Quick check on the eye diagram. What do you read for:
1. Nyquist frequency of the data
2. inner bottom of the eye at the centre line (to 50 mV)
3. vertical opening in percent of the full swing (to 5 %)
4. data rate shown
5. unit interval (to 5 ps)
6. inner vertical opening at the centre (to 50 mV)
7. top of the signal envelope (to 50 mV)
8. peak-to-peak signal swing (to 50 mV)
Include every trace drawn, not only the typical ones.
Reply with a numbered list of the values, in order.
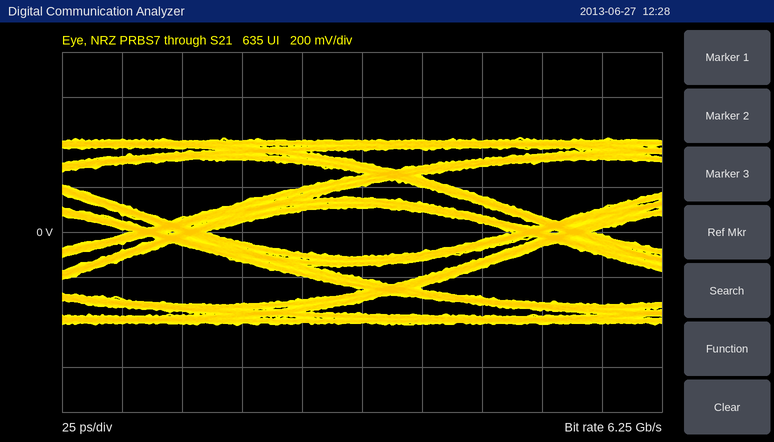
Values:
1. 3.125 GHz
2. -100 mV
3. 25 %
4. 6.25 Gb/s
5. 160 ps
6. 200 mV
7. 400 mV
8. 850 mV
